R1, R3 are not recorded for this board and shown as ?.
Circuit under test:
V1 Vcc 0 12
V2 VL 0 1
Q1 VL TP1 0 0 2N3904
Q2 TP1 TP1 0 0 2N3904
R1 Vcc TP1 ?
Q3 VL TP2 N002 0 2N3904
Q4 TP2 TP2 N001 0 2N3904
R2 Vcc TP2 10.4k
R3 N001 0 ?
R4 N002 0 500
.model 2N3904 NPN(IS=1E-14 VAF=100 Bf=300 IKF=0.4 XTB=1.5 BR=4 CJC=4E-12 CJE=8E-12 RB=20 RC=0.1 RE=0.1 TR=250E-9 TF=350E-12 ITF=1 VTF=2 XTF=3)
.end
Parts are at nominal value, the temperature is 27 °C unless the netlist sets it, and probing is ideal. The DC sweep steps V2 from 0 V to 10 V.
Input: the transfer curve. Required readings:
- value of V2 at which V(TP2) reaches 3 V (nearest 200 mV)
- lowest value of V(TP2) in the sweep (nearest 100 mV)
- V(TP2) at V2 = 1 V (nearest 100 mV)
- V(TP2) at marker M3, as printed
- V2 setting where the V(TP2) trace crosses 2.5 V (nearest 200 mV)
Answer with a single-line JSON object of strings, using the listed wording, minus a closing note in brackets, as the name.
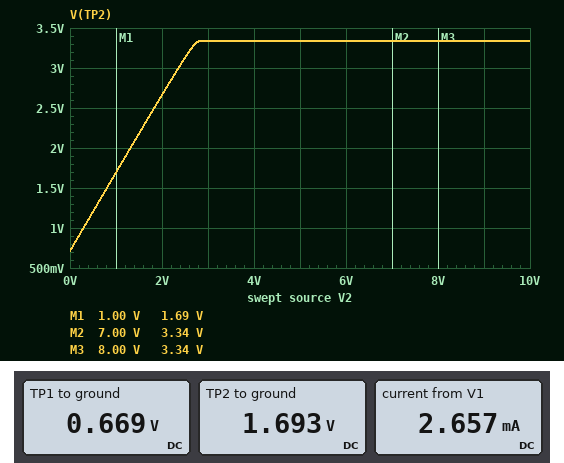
{"value of V2 at which V(TP2) reaches 3 V": "2.4 V", "lowest value of V(TP2) in the sweep": "700 mV", "V(TP2) at V2 = 1 V": "1.7 V", "V(TP2) at marker M3, as printed": "3.34 V", "V2 setting where the V(TP2) trace crosses 2.5 V": "1.8 V"}
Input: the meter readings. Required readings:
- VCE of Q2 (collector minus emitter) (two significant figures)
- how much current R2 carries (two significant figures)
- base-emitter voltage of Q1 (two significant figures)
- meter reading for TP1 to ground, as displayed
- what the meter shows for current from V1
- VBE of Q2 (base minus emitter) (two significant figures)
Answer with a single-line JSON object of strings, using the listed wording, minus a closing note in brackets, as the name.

{"VCE of Q2 (collector minus emitter)": "670 mV", "how much current R2 carries": "990 µA", "base-emitter voltage of Q1": "670 mV", "meter reading for TP1 to ground, as displayed": "0.669 V", "what the meter shows for current from V1": "2.657 mA", "VBE of Q2 (base minus emitter)": "670 mV"}
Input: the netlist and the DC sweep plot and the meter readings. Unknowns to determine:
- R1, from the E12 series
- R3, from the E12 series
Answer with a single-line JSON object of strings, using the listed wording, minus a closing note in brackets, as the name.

{"R1, from the E12 series": "6.8 kΩ", "R3, from the E12 series": "3.3 kΩ"}
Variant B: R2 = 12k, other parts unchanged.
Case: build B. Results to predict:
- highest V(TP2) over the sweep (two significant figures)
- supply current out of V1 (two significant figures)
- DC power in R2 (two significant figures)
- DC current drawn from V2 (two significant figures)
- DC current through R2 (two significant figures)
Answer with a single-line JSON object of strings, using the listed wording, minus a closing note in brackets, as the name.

{"highest V(TP2) over the sweep": "3.1 V", "supply current out of V1": "2.5 mA", "DC power in R2": "8.9 mW", "DC current drawn from V2": "3.1 mA", "DC current through R2": "860 µA"}
